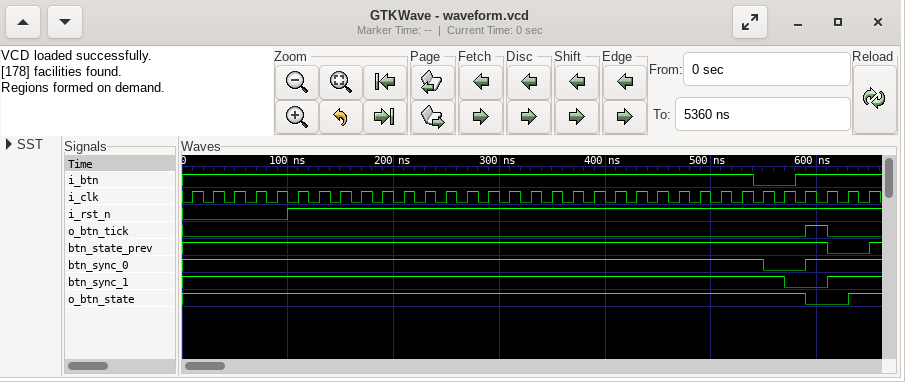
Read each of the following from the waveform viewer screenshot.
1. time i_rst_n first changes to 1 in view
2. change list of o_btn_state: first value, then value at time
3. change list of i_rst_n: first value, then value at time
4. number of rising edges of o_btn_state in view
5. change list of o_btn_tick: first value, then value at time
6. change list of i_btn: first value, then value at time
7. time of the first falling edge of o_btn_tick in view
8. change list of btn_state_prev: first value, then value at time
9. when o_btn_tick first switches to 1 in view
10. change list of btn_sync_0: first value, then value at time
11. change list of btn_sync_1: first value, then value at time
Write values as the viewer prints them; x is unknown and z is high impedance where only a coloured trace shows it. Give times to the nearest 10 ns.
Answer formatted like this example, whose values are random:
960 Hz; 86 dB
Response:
100 ns; 1, 0 at 590 ns, 1 at 630 ns; 0, 1 at 100 ns; 1; 0, 1 at 590 ns, 0 at 610 ns; 1, 0 at 540 ns, 1 at 580 ns; 610 ns; 1, 0 at 610 ns, 1 at 650 ns; 590 ns; 1, 0 at 550 ns, 1 at 590 ns; 1, 0 at 570 ns, 1 at 610 ns
